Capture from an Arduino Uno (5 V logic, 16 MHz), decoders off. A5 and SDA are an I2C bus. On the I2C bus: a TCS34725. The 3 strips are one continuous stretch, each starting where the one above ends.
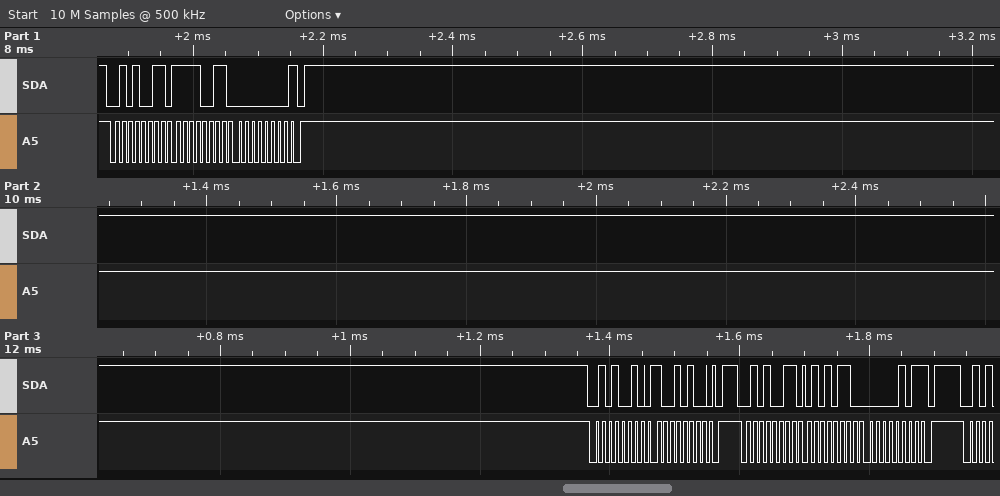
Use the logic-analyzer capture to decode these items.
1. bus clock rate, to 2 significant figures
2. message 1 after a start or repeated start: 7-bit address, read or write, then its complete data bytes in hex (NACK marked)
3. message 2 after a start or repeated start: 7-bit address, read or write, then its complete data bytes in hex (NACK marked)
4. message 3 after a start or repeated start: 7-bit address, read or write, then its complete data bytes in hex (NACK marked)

100 kHz
0x29 read: F3 00 NACK
0x29 write: 94
0x29 read: 56 05 NACK
